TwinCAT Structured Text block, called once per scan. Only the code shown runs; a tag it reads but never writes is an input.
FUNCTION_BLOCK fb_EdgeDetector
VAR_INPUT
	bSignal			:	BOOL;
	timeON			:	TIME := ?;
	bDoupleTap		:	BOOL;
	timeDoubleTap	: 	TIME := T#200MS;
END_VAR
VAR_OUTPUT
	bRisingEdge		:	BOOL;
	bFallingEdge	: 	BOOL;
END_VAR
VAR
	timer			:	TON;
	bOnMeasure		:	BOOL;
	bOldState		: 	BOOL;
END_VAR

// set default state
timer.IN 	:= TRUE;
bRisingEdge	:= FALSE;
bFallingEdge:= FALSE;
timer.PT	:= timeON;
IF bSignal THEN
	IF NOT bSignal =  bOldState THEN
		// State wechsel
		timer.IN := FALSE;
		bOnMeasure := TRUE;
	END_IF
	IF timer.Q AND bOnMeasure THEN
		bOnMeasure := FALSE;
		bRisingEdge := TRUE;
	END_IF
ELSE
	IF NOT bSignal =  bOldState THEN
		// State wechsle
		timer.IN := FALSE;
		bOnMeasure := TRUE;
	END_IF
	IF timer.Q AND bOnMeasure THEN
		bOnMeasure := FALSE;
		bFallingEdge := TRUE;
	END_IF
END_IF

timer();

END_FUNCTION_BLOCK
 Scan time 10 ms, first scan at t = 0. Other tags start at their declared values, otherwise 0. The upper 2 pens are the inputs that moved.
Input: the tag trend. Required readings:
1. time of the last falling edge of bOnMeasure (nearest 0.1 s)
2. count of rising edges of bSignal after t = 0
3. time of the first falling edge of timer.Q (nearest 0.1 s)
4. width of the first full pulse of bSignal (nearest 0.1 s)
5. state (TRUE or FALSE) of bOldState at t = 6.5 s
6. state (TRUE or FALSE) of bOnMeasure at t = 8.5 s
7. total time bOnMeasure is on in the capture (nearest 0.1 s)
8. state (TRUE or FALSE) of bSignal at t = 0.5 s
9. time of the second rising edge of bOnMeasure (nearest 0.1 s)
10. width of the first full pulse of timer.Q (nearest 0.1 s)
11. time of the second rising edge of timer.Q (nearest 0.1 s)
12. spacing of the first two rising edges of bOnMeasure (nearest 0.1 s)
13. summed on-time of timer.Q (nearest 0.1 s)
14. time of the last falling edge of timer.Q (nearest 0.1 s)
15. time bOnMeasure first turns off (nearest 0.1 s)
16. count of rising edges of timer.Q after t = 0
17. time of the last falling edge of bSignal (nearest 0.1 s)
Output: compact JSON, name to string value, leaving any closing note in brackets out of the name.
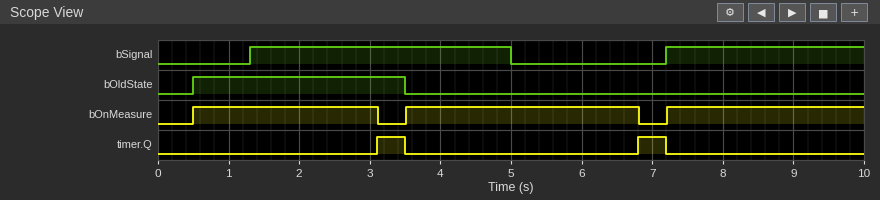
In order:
{"time of the last falling edge of bOnMeasure": "6.8 s", "count of rising edges of bSignal after t = 0": "2", "time of the first falling edge of timer.Q": "3.5 s", "width of the first full pulse of bSignal": "3.7 s", "state (TRUE or FALSE) of bOldState at t = 6.5 s": "FALSE", "state (TRUE or FALSE) of bOnMeasure at t = 8.5 s": "TRUE", "total time bOnMeasure is on in the capture": "8.7 s", "state (TRUE or FALSE) of bSignal at t = 0.5 s": "FALSE", "time of the second rising edge of bOnMeasure": "3.5 s", "width of the first full pulse of timer.Q": "0.4 s", "time of the second rising edge of timer.Q": "6.8 s", "spacing of the first two rising edges of bOnMeasure": "3.0 s", "summed on-time of timer.Q": "0.8 s", "time of the last falling edge of timer.Q": "7.2 s", "time bOnMeasure first turns off": "3.1 s", "count of rising edges of timer.Q after t = 0": "2", "time of the last falling edge of bSignal": "5.0 s"}
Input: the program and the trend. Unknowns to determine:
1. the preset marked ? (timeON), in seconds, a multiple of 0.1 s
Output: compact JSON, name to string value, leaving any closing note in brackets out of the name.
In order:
{"the preset marked ? (timeON), in seconds, a multiple of 0.1 s": "1.8 s"}
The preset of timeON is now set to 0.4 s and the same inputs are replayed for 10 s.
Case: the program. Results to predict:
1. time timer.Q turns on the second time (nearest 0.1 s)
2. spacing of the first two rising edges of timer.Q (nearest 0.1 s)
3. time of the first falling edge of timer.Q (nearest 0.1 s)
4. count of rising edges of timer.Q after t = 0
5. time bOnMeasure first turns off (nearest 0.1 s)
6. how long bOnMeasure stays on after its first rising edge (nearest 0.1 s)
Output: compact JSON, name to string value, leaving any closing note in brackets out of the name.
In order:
{"time timer.Q turns on the second time": "1.7 s", "spacing of the first two rising edges of timer.Q": "1.3 s", "time of the first falling edge of timer.Q": "0.5 s", "count of rising edges of timer.Q after t = 0": "3", "time bOnMeasure first turns off": "1.7 s", "how long bOnMeasure stays on after its first rising edge": "1.2 s"}
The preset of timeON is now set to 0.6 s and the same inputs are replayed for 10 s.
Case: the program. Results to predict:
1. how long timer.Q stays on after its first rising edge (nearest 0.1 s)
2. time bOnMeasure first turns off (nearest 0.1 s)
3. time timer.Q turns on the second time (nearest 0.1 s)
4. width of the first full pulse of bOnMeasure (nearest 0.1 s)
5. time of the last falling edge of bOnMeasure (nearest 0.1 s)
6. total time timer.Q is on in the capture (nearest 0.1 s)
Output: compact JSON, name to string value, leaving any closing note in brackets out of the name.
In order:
{"how long timer.Q stays on after its first rising edge": "1.6 s", "time bOnMeasure first turns off": "1.9 s", "time timer.Q turns on the second time": "5.6 s", "width of the first full pulse of bOnMeasure": "1.4 s", "time of the last falling edge of bOnMeasure": "5.6 s", "total time timer.Q is on in the capture": "3.2 s"}
